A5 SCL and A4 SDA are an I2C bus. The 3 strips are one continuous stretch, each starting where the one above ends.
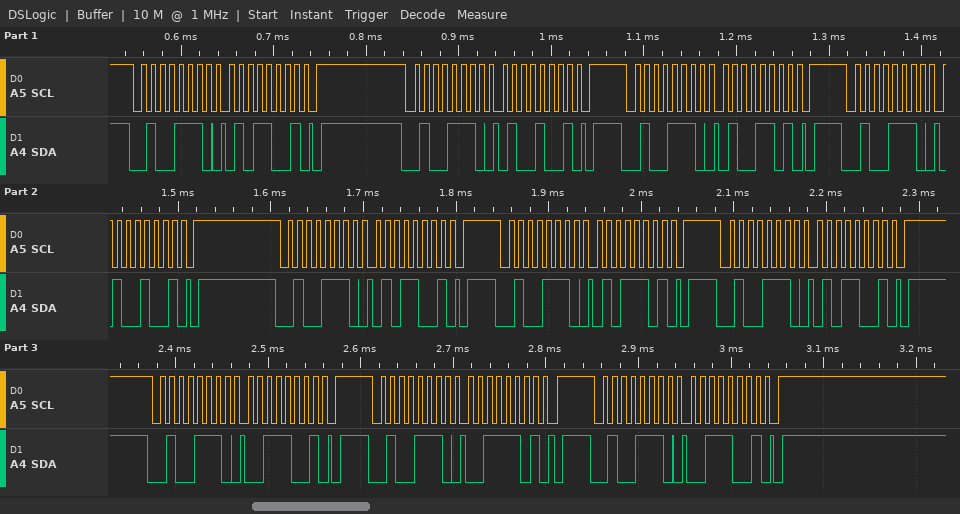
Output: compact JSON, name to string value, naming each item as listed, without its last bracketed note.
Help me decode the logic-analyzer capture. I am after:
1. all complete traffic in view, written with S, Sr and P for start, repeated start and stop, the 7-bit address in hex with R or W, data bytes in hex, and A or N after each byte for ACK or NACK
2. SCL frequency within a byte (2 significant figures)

{"all complete traffic in view, written with S, Sr and P for start, repeated start and stop, the 7-bit address in hex with R or W, data bytes in hex, and A or N after each byte for ACK or NACK": "S 27W A 59 A P S 27W A 49 A P S 27W A 4D A P S 27W A 49 A P S 27W A 59 A P S 27W A 5D A P S 27W A 59 A P S 27W A 39 A P S 27W A 3D A P S 27W A 39 A P", "SCL frequency within a byte": "100 kHz"}
